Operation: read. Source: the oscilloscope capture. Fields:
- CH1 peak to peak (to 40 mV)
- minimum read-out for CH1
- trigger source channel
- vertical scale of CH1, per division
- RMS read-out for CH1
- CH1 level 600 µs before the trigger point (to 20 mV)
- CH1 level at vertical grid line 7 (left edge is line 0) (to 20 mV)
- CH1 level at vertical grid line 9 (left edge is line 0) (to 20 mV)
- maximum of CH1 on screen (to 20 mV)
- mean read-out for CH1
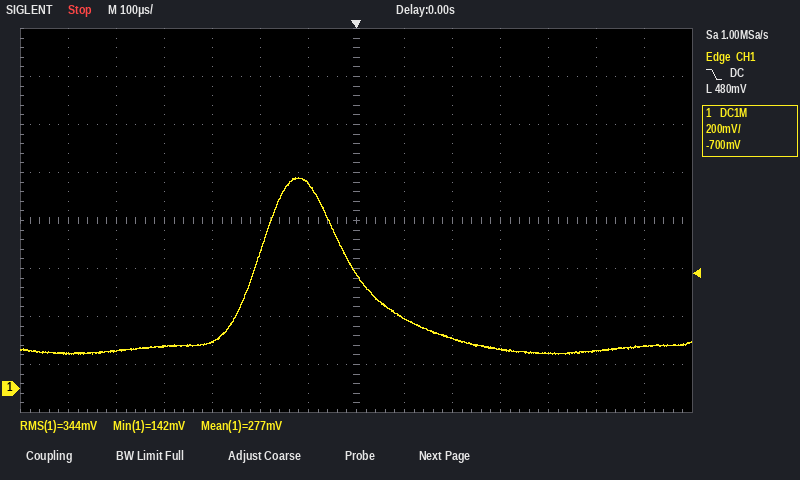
720 mV
142 mV
CH1
200 mV
344 mV
140 mV
480 mV
200 mV
880 mV
277 mV
